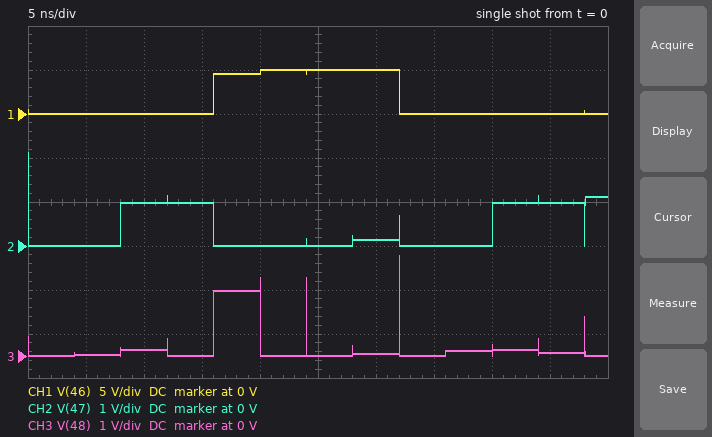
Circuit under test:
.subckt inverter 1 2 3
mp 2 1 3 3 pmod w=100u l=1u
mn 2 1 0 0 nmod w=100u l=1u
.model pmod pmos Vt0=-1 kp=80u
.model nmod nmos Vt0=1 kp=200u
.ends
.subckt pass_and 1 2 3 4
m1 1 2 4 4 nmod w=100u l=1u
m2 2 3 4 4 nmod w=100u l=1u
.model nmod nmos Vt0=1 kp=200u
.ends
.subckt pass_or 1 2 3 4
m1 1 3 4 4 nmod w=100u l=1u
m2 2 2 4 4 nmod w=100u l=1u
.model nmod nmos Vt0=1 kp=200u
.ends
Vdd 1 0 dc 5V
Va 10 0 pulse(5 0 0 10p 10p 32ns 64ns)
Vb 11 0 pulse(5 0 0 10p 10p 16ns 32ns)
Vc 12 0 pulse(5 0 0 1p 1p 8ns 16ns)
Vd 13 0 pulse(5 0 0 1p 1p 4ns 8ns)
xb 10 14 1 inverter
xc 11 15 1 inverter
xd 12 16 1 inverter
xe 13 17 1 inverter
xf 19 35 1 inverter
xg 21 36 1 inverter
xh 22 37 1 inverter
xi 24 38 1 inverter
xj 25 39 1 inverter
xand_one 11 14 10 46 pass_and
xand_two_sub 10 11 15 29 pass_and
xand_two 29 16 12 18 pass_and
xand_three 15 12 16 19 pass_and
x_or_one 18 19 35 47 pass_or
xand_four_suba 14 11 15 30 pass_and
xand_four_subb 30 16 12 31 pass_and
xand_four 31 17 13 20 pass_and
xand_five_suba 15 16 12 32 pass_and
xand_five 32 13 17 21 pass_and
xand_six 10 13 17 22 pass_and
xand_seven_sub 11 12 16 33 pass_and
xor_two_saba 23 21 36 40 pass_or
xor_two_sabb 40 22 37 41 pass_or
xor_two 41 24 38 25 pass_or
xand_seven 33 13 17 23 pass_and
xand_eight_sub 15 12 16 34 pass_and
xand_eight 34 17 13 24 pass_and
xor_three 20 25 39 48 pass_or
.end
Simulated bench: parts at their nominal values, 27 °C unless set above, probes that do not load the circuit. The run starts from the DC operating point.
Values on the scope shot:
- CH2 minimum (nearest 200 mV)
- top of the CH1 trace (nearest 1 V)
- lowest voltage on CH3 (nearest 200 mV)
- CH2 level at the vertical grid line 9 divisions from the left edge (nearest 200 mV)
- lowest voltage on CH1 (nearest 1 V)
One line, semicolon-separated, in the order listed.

0 V; 5 V; 0 V; 1.0 V; 0 V
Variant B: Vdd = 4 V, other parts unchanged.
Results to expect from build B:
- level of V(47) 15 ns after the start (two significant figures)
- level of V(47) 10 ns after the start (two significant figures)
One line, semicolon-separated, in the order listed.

960 mV; 940 mV
